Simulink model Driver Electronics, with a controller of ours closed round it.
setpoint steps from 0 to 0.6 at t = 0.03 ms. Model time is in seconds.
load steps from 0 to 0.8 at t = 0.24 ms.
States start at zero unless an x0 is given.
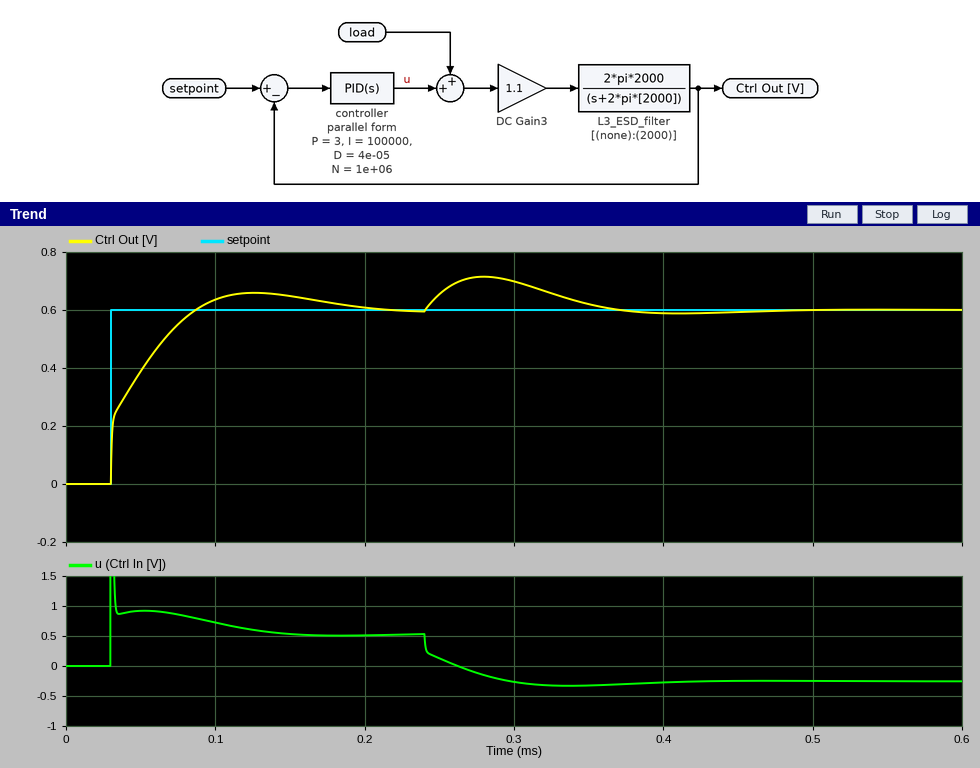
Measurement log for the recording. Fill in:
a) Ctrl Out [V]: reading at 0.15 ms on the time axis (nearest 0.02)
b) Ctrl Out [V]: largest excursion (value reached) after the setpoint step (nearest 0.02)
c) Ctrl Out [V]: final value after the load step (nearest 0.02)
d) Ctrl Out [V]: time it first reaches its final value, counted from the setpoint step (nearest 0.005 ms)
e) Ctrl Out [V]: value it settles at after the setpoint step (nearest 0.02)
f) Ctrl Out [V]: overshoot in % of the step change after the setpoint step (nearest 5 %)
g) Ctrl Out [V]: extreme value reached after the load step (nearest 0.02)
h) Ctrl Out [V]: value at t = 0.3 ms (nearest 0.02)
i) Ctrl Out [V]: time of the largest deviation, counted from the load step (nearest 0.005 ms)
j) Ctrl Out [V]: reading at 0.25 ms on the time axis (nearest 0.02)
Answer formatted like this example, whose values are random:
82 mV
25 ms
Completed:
0.64
0.66
0.60
0.055 ms
0.60
10 %
0.72
0.70
0.040 ms
0.66
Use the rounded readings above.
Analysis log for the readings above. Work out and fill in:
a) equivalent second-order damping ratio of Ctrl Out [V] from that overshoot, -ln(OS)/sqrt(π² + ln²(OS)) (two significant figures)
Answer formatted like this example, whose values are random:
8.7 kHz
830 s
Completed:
0.59
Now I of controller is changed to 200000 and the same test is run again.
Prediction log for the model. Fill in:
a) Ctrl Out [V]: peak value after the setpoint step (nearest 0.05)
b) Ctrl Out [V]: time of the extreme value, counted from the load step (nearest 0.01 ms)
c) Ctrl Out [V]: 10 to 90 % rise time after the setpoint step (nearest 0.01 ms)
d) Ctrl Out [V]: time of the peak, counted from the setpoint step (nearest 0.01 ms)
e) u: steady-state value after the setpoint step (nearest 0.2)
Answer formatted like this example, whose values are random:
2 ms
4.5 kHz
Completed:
0.70
0.03 ms
0.03 ms
0.07 ms
0.6
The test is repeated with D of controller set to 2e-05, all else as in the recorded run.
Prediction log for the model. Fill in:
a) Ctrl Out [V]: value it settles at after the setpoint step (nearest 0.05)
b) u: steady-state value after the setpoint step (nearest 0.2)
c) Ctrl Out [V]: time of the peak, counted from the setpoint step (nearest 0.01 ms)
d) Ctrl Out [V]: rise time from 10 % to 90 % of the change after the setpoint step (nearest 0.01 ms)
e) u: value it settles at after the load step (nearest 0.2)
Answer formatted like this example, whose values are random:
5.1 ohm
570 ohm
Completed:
0.60
0.6
0.08 ms
0.04 ms
-0.2
